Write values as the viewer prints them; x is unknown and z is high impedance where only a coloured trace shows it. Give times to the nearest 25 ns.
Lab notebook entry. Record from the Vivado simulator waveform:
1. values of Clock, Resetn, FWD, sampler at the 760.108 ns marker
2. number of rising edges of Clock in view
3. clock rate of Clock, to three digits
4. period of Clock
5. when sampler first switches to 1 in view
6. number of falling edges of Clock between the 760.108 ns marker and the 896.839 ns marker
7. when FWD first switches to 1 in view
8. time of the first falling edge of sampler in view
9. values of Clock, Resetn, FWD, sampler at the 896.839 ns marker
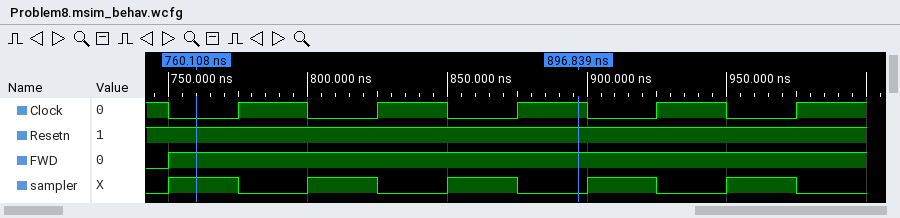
Clock=0, Resetn=1, FWD=1, sampler=1
5
20.0 MHz
50 ns
750 ns
2
750 ns
775 ns
Clock=1, Resetn=1, FWD=1, sampler=0
